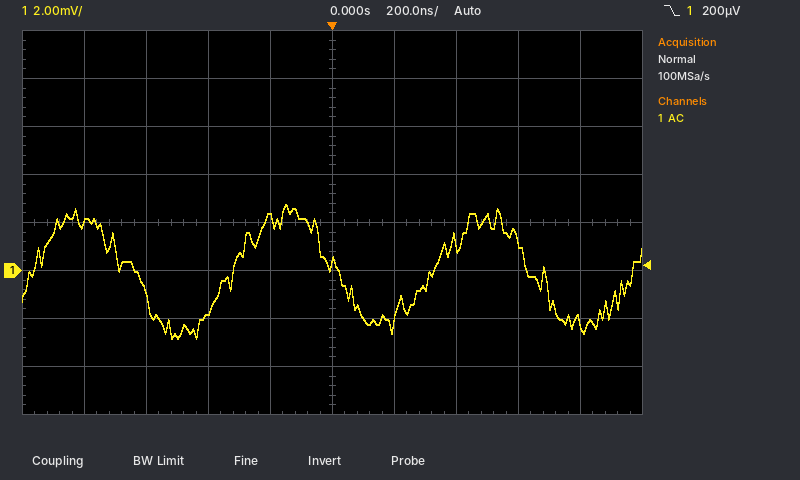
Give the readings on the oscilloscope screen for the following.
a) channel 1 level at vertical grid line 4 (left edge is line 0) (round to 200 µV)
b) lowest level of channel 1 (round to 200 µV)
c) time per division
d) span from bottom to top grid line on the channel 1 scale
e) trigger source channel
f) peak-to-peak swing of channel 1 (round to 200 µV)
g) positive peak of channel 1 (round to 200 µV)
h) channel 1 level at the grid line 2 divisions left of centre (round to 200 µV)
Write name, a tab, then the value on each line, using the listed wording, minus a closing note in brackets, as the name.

channel 1 level at vertical grid line 4 (left edge is line 0)	2.2 mV
lowest level of channel 1	-2.8 mV
time per division	200 ns
span from bottom to top grid line on the channel 1 scale	16 mV
trigger source channel	channel 1
peak-to-peak swing of channel 1	5.6 mV
positive peak of channel 1	2.8 mV
channel 1 level at the grid line 2 divisions left of centre	-1.8 mV
